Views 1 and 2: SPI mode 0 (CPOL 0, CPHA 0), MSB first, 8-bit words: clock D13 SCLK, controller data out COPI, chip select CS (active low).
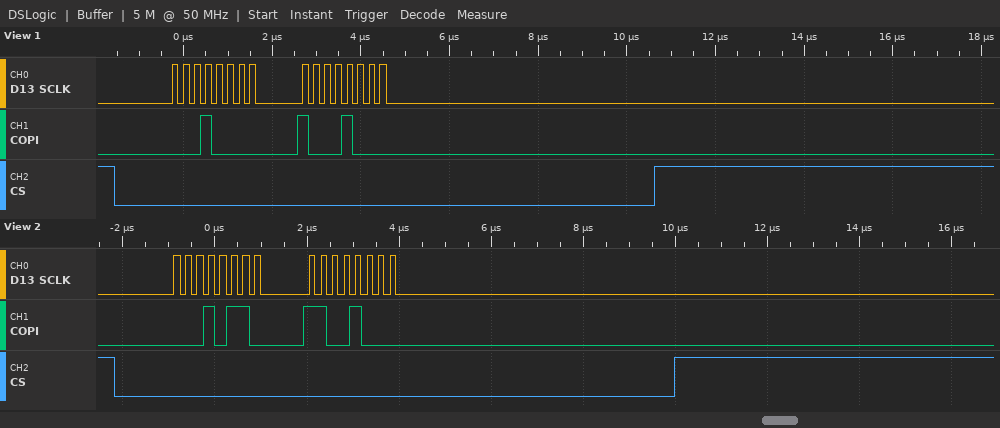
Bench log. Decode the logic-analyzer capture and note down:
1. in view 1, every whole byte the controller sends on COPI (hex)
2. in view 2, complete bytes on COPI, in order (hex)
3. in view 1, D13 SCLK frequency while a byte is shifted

10 88
16 C8
4 MHz
